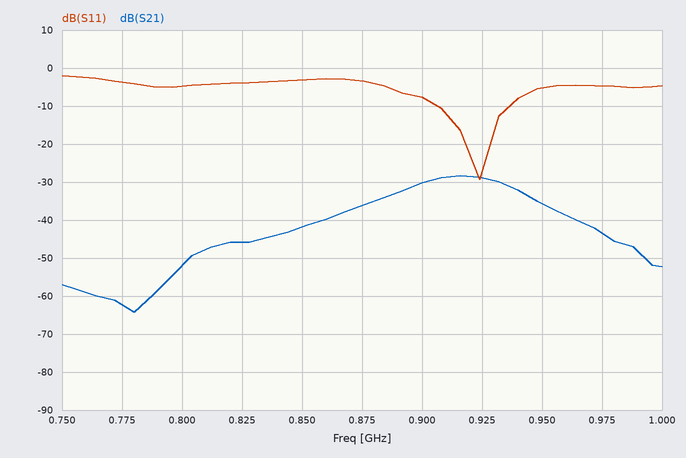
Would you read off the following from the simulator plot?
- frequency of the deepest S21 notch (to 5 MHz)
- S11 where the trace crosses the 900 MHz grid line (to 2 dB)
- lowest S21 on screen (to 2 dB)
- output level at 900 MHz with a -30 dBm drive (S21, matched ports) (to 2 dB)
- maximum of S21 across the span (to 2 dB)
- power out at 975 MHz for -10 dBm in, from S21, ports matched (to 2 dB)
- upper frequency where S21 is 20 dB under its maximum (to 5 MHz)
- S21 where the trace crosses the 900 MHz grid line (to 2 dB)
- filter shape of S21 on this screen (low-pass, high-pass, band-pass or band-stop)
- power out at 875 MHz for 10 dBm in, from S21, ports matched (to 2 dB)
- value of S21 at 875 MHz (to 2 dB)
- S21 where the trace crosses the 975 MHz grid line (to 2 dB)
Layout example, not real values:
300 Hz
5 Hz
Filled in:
780 MHz
-8 dB
-64 dB
-60 dBm
-28 dB
-54 dBm
990 MHz
-30 dB
band-pass
-26 dBm
-36 dB
-44 dB
